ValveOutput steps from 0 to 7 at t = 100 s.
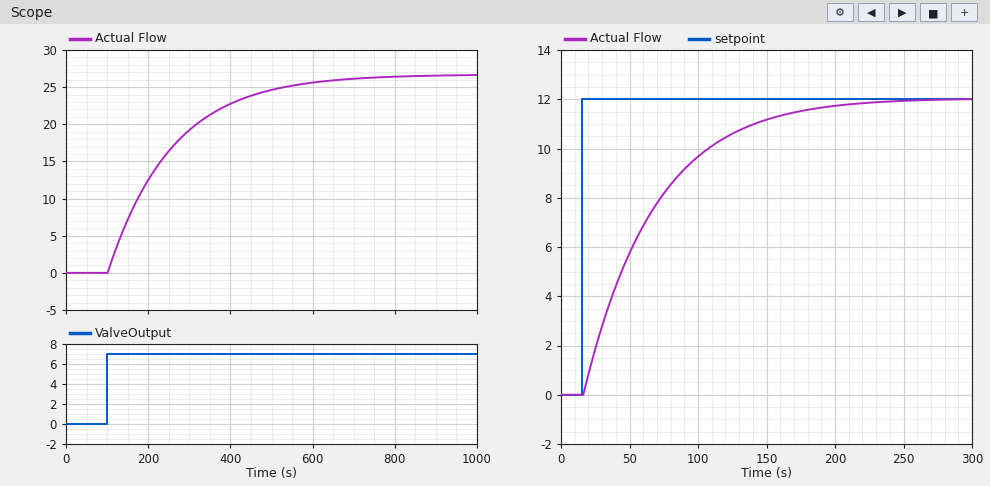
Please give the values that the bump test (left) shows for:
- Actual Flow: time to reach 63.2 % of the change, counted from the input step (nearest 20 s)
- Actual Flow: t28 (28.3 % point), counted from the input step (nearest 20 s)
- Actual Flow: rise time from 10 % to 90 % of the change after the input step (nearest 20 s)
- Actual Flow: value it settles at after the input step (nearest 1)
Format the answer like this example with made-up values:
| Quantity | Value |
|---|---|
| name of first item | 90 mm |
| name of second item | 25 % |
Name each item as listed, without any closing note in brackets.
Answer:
| Quantity | Value |
|---|---|
| Actual Flow: time to reach 63.2 % of the change, counted from the input step | 160 s |
| Actual Flow: t28 (28.3 % point), counted from the input step | 60 s |
| Actual Flow: rise time from 10 % to 90 % of the change after the input step | 340 s |
| Actual Flow: value it settles at after the input step | 27 |
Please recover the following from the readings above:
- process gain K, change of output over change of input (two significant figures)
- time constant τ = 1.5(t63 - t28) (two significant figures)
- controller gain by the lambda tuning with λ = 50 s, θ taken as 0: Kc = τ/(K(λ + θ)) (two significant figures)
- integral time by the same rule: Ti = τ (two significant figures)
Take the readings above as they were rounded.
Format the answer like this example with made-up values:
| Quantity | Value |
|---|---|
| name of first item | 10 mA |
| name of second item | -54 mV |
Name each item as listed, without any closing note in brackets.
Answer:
| Quantity | Value |
|---|---|
| process gain K, change of output over change of input | 3.9 |
| time constant τ = 1.5(t63 - t28) | 150 s |
| controller gain by the lambda tuning with λ = 50 s, θ taken as 0: Kc = τ/(K(λ + θ)) | 0.77 |
| integral time by the same rule: Ti = τ | 150 s |
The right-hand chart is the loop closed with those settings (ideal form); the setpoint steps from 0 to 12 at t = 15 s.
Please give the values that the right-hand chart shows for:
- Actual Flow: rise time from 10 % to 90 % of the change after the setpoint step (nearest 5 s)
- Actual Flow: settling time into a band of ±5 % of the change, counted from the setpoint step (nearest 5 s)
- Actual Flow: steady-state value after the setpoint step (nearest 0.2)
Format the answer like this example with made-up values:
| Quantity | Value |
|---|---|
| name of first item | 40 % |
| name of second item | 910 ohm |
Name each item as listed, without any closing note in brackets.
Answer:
| Quantity | Value |
|---|---|
| Actual Flow: rise time from 10 % to 90 % of the change after the setpoint step | 110 s |
| Actual Flow: settling time into a band of ±5 % of the change, counted from the setpoint step | 150 s |
| Actual Flow: steady-state value after the setpoint step | 12.0 |
